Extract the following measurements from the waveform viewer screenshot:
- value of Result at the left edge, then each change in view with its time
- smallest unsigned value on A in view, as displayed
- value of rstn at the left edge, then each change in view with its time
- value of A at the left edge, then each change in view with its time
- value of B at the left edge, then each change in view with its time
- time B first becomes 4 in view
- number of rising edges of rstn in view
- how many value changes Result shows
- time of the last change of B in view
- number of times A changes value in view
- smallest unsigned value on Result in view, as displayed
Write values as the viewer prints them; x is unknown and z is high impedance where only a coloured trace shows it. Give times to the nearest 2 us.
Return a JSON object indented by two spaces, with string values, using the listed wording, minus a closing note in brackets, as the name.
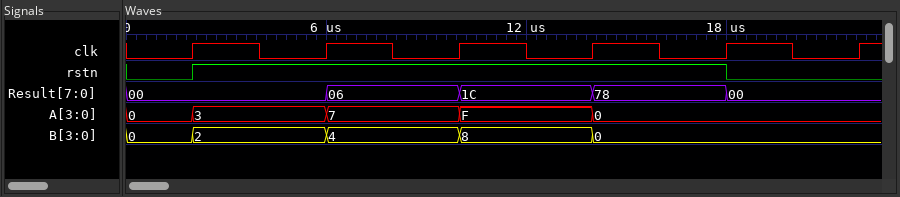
{
  "value of Result at the left edge, then each change in view with its time": "00, 06 at 6 us, 1C at 10 us, 78 at 14 us, 00 at 18 us",
  "smallest unsigned value on A in view, as displayed": "0",
  "value of rstn at the left edge, then each change in view with its time": "0, 1 at 2 us, 0 at 18 us",
  "value of A at the left edge, then each change in view with its time": "0, 3 at 2 us, 7 at 6 us, F at 10 us, 0 at 14 us",
  "value of B at the left edge, then each change in view with its time": "0, 2 at 2 us, 4 at 6 us, 8 at 10 us, 0 at 14 us",
  "time B first becomes 4 in view": "6 us",
  "number of rising edges of rstn in view": "1",
  "how many value changes Result shows": "4",
  "time of the last change of B in view": "14 us",
  "number of times A changes value in view": "4",
  "smallest unsigned value on Result in view, as displayed": "00"
}
